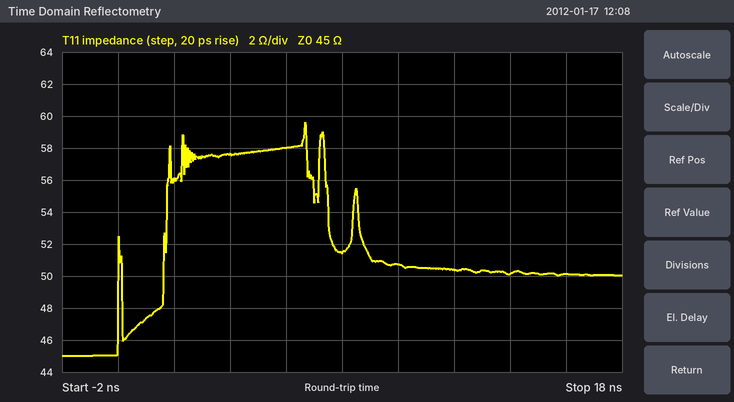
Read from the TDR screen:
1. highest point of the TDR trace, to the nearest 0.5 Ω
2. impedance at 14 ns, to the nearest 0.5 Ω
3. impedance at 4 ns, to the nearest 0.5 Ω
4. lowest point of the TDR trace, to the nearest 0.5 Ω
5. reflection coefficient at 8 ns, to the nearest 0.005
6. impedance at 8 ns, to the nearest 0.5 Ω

59.5 Ω
50.0 Ω
57.5 Ω
45.0 Ω
+0.065
51.5 Ω
